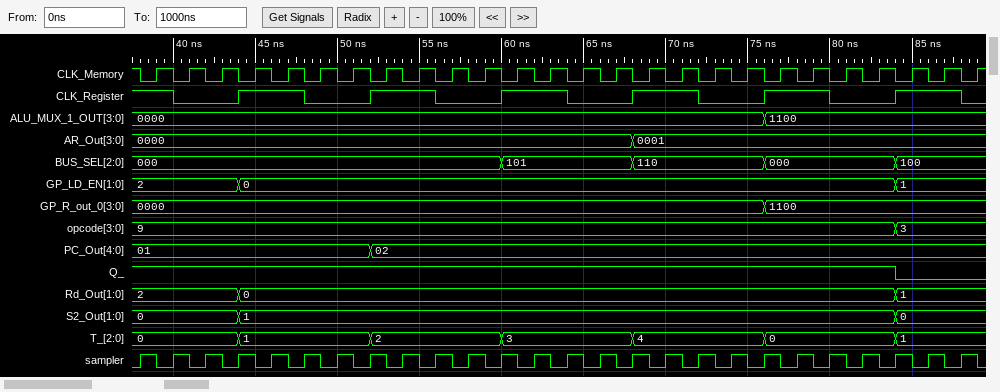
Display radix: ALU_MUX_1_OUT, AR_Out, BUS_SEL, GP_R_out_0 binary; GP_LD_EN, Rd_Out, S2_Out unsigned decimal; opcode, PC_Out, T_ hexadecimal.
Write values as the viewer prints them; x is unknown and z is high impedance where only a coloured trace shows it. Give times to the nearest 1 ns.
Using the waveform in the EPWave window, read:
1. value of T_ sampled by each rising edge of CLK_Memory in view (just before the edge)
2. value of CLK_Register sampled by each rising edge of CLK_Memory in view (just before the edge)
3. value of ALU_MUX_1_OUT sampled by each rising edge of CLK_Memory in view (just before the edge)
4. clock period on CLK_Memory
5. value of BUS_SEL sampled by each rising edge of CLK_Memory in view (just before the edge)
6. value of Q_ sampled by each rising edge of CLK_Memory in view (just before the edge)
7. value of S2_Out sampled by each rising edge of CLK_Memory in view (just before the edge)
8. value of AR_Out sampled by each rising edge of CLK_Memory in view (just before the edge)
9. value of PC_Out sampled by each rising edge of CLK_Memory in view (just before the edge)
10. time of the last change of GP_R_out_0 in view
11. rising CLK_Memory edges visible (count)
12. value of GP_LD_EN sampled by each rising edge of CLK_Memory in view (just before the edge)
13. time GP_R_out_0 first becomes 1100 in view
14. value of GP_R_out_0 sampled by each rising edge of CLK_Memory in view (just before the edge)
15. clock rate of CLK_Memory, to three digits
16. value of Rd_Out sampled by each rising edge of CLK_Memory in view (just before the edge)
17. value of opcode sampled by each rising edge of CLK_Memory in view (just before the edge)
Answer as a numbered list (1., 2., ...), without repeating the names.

1. 0, 0, 0, 1, 1, 1, 1, 2, 2, 2, 2, 3, 3, 3, 3, 4, 4, 4, 4, 0, 0, 0, 0, 1, 1, 1
2. 1 0 0 1 1 0 0 1 1 0 0 1 1 0 0 1 1 0 0 1 1 0 0 1 1 0
3. 0000, 0000, 0000, 0000, 0000, 0000, 0000, 0000, 0000, 0000, 0000, 0000, 0000, 0000, 0000, 0000, 0000, 0000, 0000, 1100, 1100, 1100, 1100, 1100, 1100, 1100
4. 2 ns
5. 000, 000, 000, 000, 000, 000, 000, 000, 000, 000, 000, 101, 101, 101, 101, 110, 110, 110, 110, 000, 000, 000, 000, 100, 100, 100
6. 1 1 1 1 1 1 1 1 1 1 1 1 1 1 1 1 1 1 1 1 1 1 1 0 0 0
7. 0, 0, 0, 1, 1, 1, 1, 1, 1, 1, 1, 1, 1, 1, 1, 1, 1, 1, 1, 1, 1, 1, 1, 0, 0, 0
8. 0000, 0000, 0000, 0000, 0000, 0000, 0000, 0000, 0000, 0000, 0000, 0000, 0000, 0000, 0000, 0001, 0001, 0001, 0001, 0001, 0001, 0001, 0001, 0001, 0001, 0001
9. 01, 01, 01, 01, 01, 01, 01, 02, 02, 02, 02, 02, 02, 02, 02, 02, 02, 02, 02, 02, 02, 02, 02, 02, 02, 02
10. 76 ns
11. 26
12. 2, 2, 2, 0, 0, 0, 0, 0, 0, 0, 0, 0, 0, 0, 0, 0, 0, 0, 0, 0, 0, 0, 0, 1, 1, 1
13. 76 ns
14. 0000, 0000, 0000, 0000, 0000, 0000, 0000, 0000, 0000, 0000, 0000, 0000, 0000, 0000, 0000, 0000, 0000, 0000, 0000, 1100, 1100, 1100, 1100, 1100, 1100, 1100
15. 500 MHz
16. 2, 2, 2, 0, 0, 0, 0, 0, 0, 0, 0, 0, 0, 0, 0, 0, 0, 0, 0, 0, 0, 0, 0, 1, 1, 1
17. 9, 9, 9, 9, 9, 9, 9, 9, 9, 9, 9, 9, 9, 9, 9, 9, 9, 9, 9, 9, 9, 9, 9, 3, 3, 3
